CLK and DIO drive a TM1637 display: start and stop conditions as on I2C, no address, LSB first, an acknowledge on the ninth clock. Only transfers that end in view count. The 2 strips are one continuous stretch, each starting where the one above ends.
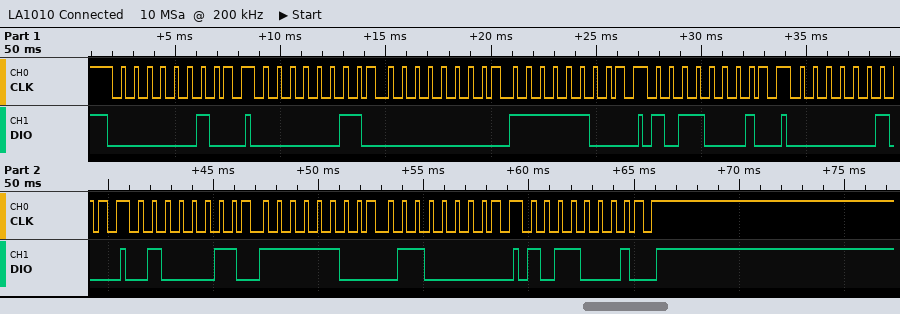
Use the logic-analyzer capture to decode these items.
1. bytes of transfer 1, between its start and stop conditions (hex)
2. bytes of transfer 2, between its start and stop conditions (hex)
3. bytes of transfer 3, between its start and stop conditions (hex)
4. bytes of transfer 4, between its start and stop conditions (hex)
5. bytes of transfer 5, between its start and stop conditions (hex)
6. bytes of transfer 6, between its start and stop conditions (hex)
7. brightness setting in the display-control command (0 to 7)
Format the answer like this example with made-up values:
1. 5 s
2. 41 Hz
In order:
1. 40
2. C0 00 3F
3. 8D
4. 40
5. C2 3F 06
6. 8D
7. 5
